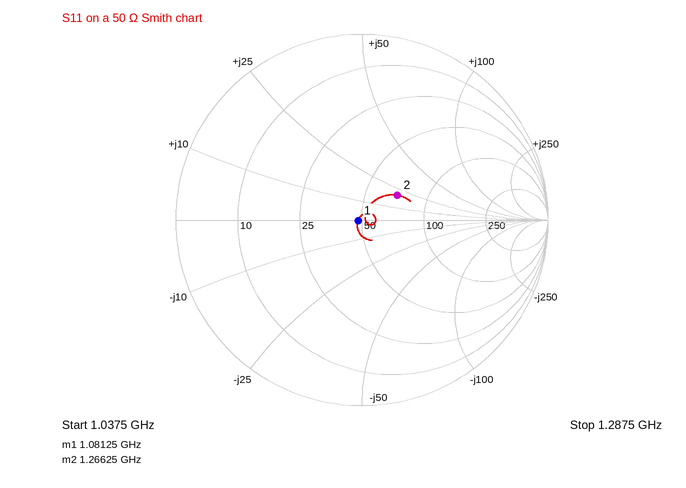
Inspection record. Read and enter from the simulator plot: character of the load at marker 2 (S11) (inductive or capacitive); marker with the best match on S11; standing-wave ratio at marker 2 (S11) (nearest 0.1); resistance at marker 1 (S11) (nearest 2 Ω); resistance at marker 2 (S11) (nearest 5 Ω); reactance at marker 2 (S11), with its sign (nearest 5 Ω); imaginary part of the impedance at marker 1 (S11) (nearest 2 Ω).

inductive
marker 1
1.6
48 Ω
70 Ω
+20 Ω
0 Ω
